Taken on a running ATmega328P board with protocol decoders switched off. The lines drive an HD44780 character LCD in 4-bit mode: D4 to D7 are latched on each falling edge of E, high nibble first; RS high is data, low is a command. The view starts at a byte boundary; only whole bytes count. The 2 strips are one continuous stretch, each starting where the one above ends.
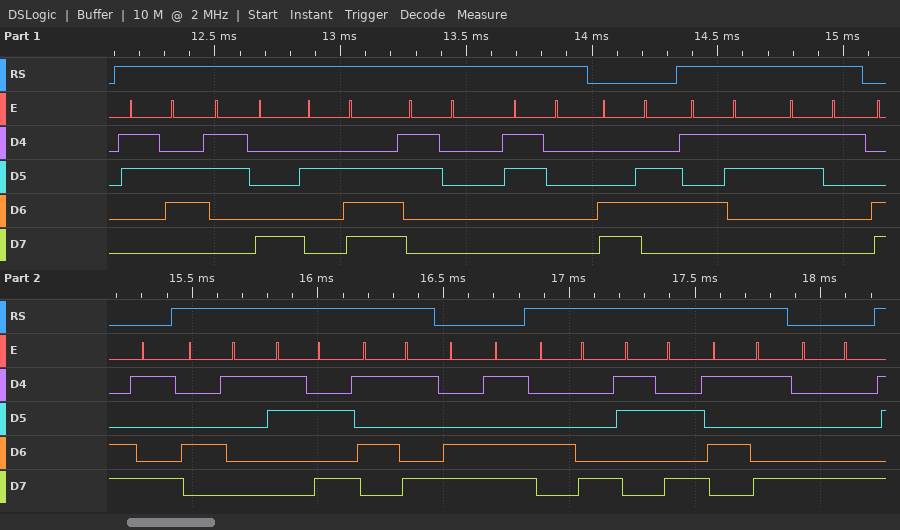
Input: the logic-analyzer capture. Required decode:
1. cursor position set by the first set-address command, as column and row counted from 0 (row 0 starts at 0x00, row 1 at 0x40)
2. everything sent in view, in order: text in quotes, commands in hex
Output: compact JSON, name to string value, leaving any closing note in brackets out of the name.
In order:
{"cursor position set by the first set-address command, as column and row counted from 0": "column 6, row 1", "everything sent in view, in order: text in quotes, commands in hex": "\"68.00\" 0xC6 \"S1\" 0xC9 \"A:Y\" 0xCD \"H:Y\" 0x88"}
